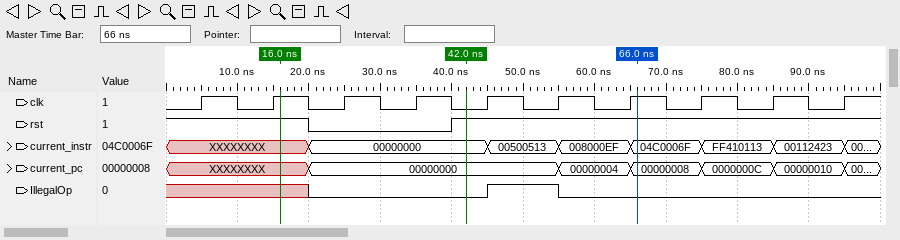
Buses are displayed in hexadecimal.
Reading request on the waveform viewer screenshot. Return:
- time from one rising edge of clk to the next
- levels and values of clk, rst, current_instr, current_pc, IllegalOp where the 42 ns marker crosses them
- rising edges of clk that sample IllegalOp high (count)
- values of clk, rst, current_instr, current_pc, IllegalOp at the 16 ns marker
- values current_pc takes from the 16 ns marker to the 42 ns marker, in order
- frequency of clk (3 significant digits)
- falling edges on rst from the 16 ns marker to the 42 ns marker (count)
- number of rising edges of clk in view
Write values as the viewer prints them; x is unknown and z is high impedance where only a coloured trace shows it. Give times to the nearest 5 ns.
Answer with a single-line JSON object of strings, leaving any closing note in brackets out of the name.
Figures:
{"time from one rising edge of clk to the next": "10 ns", "levels and values of clk, rst, current_instr, current_pc, IllegalOp where the 42 ns marker crosses them": "clk=0, rst=1, current_instr=00000000, current_pc=00000000, IllegalOp=0", "rising edges of clk that sample IllegalOp high": "1", "values of clk, rst, current_instr, current_pc, IllegalOp at the 16 ns marker": "clk=1, rst=1, current_instr=XXXXXXXX, current_pc=XXXXXXXX, IllegalOp=x", "values current_pc takes from the 16 ns marker to the 42 ns marker, in order": "XXXXXXXX, 00000000", "frequency of clk": "100 MHz", "falling edges on rst from the 16 ns marker to the 42 ns marker": "1", "number of rising edges of clk in view": "10"}
